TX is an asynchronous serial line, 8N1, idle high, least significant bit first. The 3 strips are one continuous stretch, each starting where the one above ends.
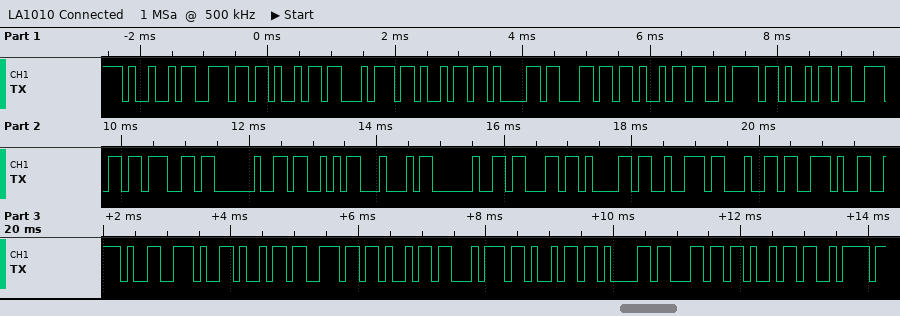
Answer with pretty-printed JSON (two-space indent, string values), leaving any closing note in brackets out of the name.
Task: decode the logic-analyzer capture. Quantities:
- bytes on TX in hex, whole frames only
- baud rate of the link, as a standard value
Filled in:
{
  "bytes on TX in hex, whole frames only": "49 6E 69 74 69 61 6C 69 7A 69 6E 67 20 53 44 20 63 61 72 64 2E 2E 2E 69 6E 69 74 69 61 6C 69 7A",
  "baud rate of the link, as a standard value": "9600 baud"
}
